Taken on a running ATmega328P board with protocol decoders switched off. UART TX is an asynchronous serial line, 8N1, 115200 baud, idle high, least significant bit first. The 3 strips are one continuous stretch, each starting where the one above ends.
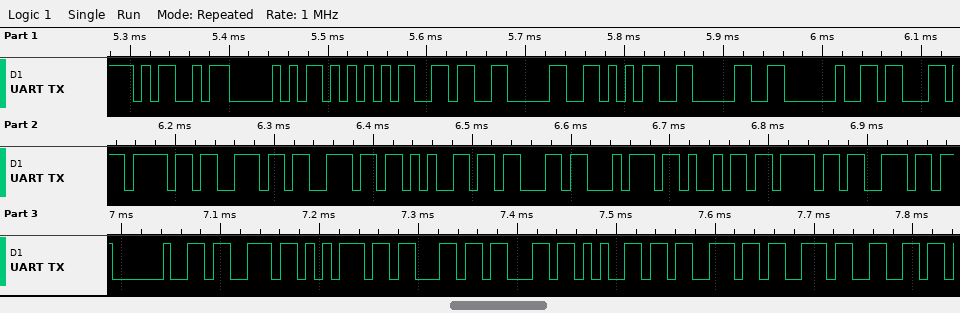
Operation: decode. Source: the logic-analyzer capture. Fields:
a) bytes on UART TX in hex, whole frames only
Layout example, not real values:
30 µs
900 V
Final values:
0x4D 0x50 0x55 0x36 0x30 0x35 0x30 0x20 0x63 0x6F 0x6E 0x6E 0x65 0x63 0x74 0x69 0x6F 0x6E 0x20 0x73 0x75 0x63 0x63 0x65 0x73 0x73 0x66
